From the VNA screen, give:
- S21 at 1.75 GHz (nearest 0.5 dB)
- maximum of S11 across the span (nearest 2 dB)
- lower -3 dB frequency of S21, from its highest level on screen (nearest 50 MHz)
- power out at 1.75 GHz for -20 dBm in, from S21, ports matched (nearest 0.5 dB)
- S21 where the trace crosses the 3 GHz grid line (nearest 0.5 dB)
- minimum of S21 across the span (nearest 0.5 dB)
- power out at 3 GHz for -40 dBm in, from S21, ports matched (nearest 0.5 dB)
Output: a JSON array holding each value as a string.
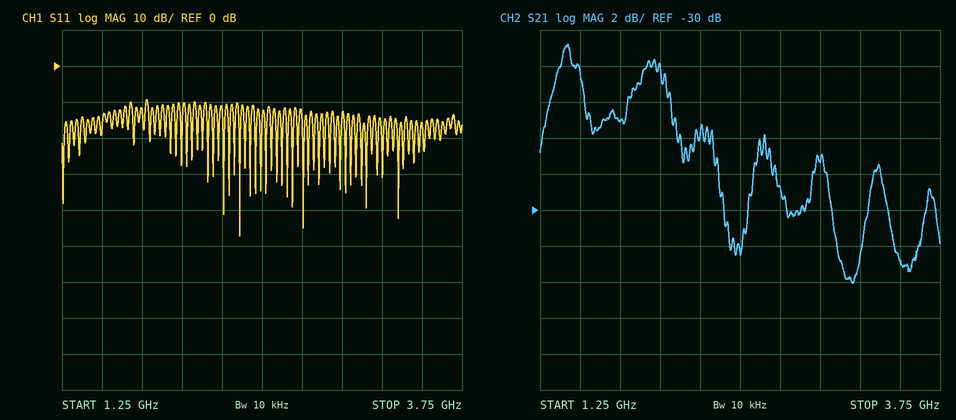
["-25.0 dB", "-10 dB", "1.30 GHz", "-45.0 dBm", "-27.5 dB", "-34.0 dB", "-67.5 dBm"]
